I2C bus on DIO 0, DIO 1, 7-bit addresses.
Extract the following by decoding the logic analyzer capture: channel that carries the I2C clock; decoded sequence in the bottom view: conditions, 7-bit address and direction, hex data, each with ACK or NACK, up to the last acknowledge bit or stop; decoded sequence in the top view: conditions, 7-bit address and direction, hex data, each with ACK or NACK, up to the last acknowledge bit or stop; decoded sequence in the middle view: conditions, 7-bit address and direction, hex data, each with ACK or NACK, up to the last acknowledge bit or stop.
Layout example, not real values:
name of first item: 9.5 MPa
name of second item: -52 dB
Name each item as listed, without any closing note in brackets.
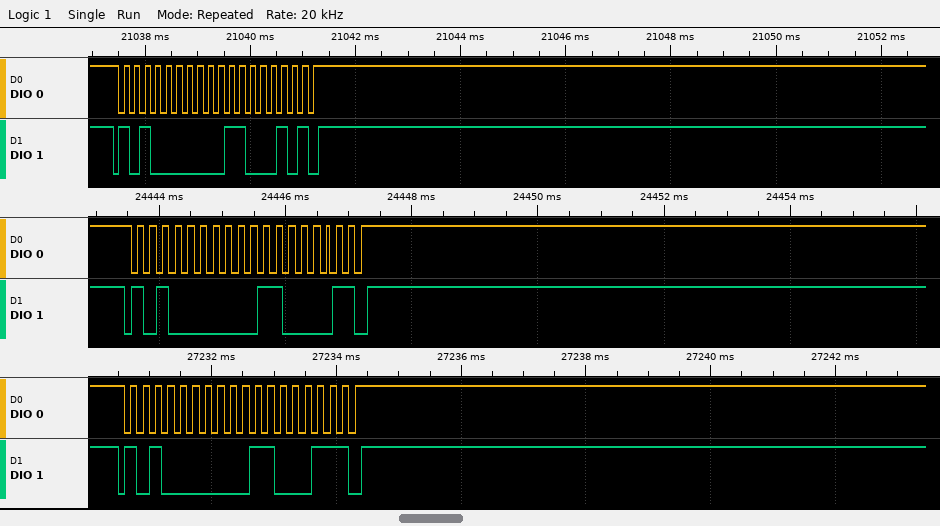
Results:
channel that carries the I2C clock: DIO 0
decoded sequence in the bottom view: conditions, 7-bit address and direction, hex data, each with ACK or NACK, up to the last acknowledge bit or stop: start, address 50 write ACK, 63 NACK, stop
decoded sequence in the top view: conditions, 7-bit address and direction, hex data, each with ACK or NACK, up to the last acknowledge bit or stop: start, address 50 write ACK, 62 NACK, stop
decoded sequence in the middle view: conditions, 7-bit address and direction, hex data, each with ACK or NACK, up to the last acknowledge bit or stop: start, address 50 write ACK, 61 NACK, stop
